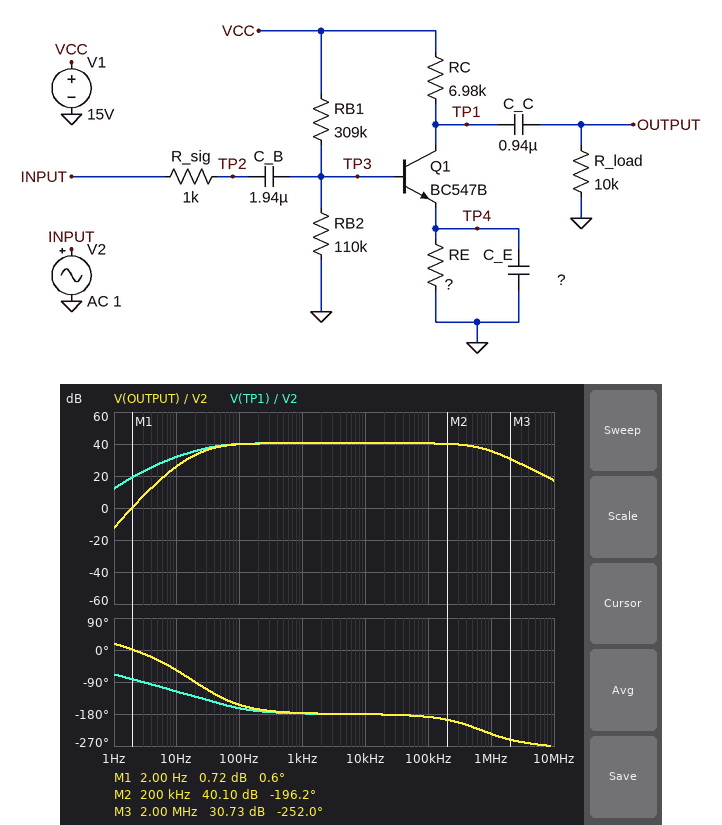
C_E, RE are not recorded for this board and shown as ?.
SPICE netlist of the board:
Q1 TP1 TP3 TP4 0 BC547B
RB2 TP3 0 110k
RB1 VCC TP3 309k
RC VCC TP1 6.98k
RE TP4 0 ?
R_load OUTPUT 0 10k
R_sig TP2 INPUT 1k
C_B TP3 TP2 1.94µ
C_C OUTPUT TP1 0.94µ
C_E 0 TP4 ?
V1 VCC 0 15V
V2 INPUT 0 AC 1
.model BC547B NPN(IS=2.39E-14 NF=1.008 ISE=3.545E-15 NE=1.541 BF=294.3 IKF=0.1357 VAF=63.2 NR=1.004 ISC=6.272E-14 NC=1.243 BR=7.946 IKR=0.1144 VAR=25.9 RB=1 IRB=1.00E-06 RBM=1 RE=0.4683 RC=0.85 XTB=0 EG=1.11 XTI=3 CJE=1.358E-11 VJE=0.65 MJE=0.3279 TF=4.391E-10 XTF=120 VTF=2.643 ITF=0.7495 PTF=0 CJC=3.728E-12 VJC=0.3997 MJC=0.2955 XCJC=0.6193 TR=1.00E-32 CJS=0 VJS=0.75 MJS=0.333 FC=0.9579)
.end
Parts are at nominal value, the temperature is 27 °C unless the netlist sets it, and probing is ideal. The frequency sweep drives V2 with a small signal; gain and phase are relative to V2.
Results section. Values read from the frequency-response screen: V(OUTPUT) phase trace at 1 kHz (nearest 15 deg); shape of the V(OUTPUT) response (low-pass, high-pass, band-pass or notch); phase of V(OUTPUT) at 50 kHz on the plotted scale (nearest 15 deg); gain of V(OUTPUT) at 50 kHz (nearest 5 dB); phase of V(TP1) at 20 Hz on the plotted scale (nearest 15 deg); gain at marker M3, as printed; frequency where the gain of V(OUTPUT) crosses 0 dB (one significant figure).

-180 deg
band-pass
-180 deg
40 dB
-135 deg
30.73 dB
2 Hz
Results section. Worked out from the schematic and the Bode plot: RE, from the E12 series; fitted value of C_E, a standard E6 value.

3.9 kΩ
150 µF
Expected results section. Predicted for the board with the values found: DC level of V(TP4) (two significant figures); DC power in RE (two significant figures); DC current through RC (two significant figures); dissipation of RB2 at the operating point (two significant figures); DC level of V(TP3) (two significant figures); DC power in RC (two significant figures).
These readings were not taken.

3.1 V
2.5 mW
790 µA
130 µW
3.7 V
4.4 mW
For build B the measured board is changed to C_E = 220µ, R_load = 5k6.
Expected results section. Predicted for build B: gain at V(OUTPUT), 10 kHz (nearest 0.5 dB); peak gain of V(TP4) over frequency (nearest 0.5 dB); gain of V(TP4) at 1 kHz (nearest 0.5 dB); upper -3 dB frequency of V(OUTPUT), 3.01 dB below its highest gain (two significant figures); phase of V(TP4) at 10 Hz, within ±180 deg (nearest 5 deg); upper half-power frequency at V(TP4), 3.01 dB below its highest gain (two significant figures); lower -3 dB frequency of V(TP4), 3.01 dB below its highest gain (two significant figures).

38.0 dB
-3.5 dB
-34.5 dB
850 kHz
-15 deg
28 Hz
730 mHz
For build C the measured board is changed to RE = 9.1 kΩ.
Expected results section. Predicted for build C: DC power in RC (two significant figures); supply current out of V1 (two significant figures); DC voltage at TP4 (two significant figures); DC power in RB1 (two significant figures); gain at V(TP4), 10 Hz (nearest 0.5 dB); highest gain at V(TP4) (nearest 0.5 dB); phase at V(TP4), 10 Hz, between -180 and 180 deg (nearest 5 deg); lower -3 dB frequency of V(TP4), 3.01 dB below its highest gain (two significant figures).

880 µW
390 µA
3.2 V
400 µW
-3.5 dB
-2.5 dB
-25 deg
750 mHz
